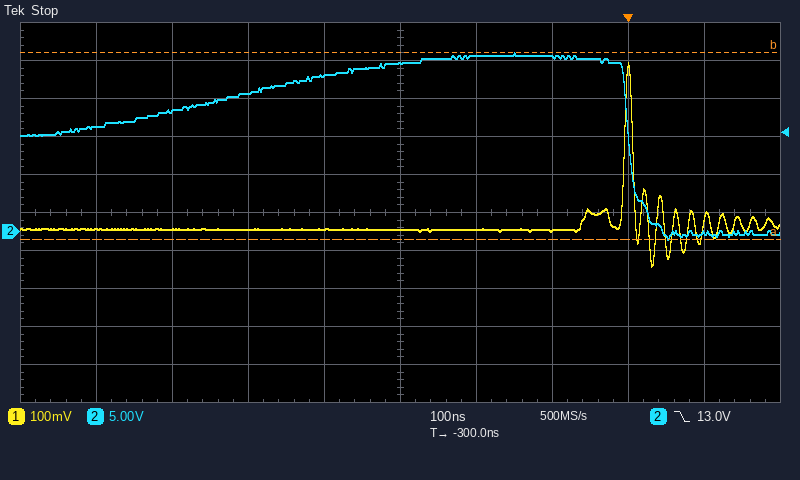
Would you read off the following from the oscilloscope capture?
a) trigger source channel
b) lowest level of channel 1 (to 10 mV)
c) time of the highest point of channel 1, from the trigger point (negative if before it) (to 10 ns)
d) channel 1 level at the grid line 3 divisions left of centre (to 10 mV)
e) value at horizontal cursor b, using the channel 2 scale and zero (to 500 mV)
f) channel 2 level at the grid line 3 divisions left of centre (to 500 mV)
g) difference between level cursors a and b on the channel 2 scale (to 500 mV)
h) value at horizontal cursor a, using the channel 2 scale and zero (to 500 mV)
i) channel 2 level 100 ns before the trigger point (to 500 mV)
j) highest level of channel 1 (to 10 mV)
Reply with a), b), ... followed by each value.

a) channel 2
b) -90 mV
c) 0 ns
d) 10 mV
e) 23.5 V
f) 16.0 V
g) 24.5 V
h) -1.0 V
i) 23.0 V
j) 440 mV
